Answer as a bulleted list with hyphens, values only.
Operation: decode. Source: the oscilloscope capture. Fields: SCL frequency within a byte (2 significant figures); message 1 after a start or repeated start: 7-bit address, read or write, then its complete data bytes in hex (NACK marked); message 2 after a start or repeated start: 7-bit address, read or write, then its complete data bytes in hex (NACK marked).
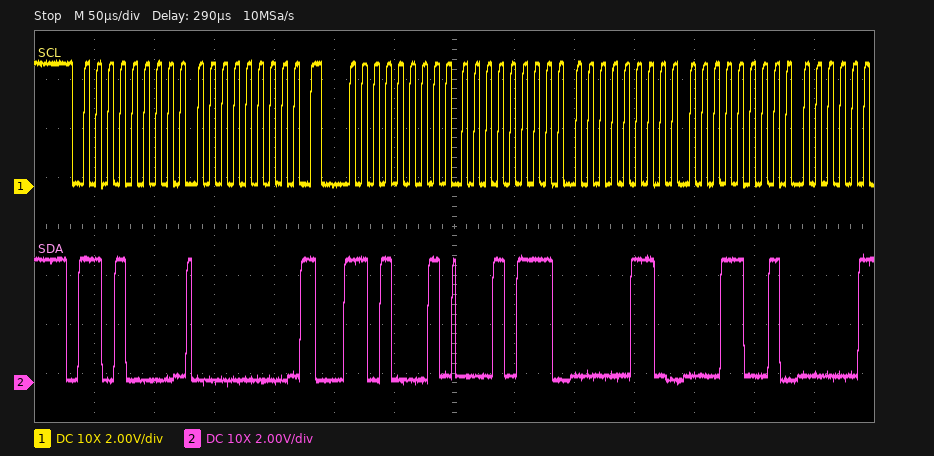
- 100 kHz
- 0x68 write: 00
- 0x68 read: 17 06 19
